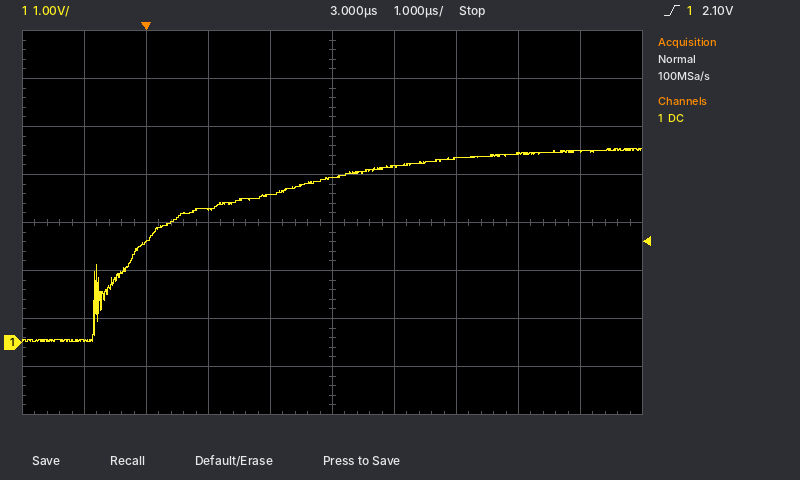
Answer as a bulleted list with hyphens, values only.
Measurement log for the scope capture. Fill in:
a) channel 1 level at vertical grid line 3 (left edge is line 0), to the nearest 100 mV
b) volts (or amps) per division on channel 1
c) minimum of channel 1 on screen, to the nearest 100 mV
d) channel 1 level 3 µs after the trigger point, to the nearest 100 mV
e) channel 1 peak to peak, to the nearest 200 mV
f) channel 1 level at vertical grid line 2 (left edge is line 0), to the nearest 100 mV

- 2.8 V
- 1 V
- 0.0 V
- 3.4 V
- 4.0 V
- 2.1 V
